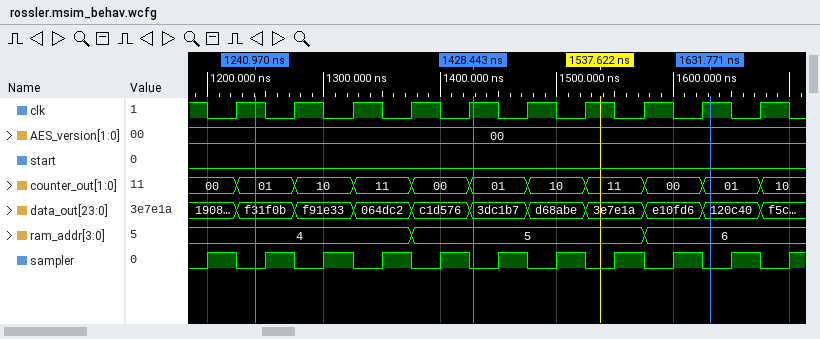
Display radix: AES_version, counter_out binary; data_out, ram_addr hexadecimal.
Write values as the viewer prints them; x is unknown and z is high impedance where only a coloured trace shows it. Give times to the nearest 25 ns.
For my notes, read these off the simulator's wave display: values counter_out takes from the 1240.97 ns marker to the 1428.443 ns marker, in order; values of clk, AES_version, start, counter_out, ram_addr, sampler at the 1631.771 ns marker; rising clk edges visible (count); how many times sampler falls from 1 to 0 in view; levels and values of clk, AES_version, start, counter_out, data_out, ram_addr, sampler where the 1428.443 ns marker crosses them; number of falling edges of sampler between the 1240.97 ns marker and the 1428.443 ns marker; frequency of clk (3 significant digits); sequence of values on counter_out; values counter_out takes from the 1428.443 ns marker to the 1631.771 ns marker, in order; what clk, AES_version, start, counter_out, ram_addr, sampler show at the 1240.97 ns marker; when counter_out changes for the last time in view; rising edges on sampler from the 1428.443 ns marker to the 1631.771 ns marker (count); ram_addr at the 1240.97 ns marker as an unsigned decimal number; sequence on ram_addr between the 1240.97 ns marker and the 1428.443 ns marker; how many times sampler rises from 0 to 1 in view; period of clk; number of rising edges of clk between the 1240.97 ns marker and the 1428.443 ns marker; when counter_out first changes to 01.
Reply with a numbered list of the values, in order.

1. 01, 10, 11, 00, 01
2. clk=1, AES_version=00, start=0, counter_out=01, ram_addr=6, sampler=0
3. 10
4. 10
5. clk=1, AES_version=00, start=0, counter_out=01, data_out=3dc1b7, ram_addr=5, sampler=0
6. 4
7. 20.0 MHz
8. 00, 01, 10, 11, 00, 01, 10, 11, 00, 01, 10
9. 01, 10, 11, 00, 01
10. clk=1, AES_version=00, start=0, counter_out=01, ram_addr=4, sampler=0
11. 1675 ns
12. 4
13. 4
14. 4, 5
15. 11
16. 50 ns
17. 4
18. 1225 ns
